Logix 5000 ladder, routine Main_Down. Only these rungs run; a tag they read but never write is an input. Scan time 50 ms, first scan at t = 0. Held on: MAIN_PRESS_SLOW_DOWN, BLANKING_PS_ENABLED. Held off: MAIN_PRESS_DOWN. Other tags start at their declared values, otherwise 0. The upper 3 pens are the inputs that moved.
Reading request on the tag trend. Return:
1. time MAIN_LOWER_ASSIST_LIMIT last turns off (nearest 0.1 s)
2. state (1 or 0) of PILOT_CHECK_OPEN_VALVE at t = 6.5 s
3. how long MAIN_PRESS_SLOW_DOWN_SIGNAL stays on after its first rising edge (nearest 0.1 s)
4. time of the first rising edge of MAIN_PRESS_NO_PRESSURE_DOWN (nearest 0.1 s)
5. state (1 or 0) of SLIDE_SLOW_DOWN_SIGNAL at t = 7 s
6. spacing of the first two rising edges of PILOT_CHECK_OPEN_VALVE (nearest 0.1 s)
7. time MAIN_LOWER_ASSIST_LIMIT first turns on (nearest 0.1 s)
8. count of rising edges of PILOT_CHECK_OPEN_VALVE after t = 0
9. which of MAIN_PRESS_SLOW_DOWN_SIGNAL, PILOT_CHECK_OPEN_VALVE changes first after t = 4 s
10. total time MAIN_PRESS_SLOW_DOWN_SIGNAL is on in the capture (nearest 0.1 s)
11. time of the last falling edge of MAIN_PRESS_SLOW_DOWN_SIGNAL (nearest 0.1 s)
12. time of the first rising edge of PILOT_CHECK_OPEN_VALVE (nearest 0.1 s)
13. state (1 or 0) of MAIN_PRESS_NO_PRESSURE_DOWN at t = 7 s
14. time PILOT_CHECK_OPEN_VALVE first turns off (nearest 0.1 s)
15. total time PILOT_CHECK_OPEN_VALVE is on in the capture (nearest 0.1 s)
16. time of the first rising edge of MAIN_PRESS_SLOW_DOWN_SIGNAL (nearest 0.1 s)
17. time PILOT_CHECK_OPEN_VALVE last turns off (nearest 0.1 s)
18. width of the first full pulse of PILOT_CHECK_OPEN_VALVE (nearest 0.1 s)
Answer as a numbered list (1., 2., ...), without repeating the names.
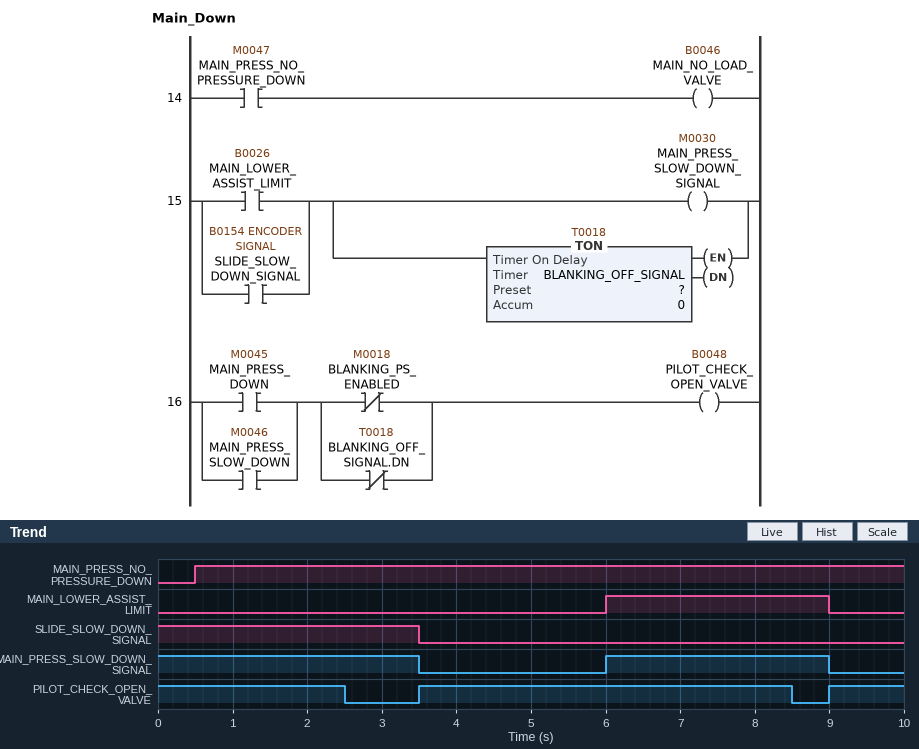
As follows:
1. 9.0 s
2. 1
3. 3.0 s
4. 0.5 s
5. 0
6. 5.5 s
7. 6.0 s
8. 2
9. MAIN_PRESS_SLOW_DOWN_SIGNAL
10. 6.5 s
11. 9.0 s
12. 3.5 s
13. 1
14. 2.5 s
15. 8.5 s
16. 6.0 s
17. 8.5 s
18. 5.0 s
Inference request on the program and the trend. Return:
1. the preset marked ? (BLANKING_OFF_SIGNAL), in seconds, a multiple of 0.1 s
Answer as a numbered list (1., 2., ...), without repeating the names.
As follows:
1. 2.5 s
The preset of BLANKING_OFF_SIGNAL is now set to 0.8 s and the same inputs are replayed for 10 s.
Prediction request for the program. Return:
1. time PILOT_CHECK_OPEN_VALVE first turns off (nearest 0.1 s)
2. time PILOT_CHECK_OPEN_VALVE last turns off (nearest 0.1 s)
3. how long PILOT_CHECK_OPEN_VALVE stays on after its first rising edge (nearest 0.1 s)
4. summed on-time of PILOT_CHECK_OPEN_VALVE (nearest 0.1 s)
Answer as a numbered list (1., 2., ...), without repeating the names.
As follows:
1. 0.8 s
2. 6.8 s
3. 3.3 s
4. 5.1 s
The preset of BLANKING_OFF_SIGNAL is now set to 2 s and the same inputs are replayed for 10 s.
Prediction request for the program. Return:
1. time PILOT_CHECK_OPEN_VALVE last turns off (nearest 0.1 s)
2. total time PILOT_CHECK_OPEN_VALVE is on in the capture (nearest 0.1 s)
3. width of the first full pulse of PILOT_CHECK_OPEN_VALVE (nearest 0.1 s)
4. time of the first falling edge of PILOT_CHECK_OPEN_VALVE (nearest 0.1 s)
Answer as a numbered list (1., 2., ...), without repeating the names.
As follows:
1. 8.0 s
2. 7.5 s
3. 4.5 s
4. 2.0 s
